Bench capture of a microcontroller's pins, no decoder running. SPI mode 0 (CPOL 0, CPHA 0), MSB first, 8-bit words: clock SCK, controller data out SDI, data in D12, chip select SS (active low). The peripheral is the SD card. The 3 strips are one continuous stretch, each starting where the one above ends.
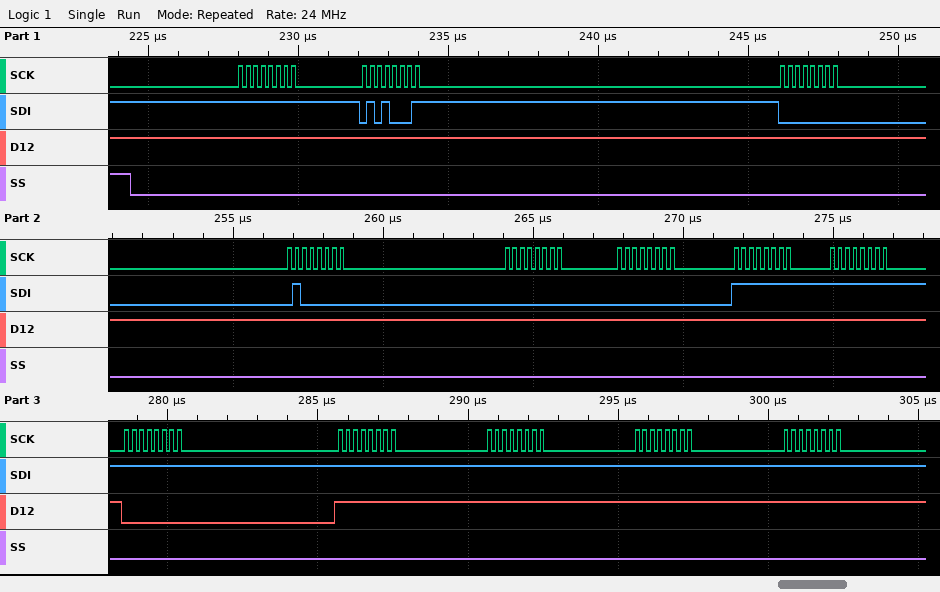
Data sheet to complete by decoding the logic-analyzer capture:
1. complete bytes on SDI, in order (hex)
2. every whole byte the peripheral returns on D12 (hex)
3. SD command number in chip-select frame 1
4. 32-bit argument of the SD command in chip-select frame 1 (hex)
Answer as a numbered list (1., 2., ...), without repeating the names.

1. 0xFF 0x51 0x00 0x40 0x00 0x00 0xFF 0xFF 0xFF 0xFF 0xFF 0xFF 0xFF
2. 0xFF 0xFF 0xFF 0xFF 0xFF 0xFF 0xFF 0xFF 0x00 0xFF 0xFF 0xFF 0xFF
3. CMD17
4. 0x00400000
